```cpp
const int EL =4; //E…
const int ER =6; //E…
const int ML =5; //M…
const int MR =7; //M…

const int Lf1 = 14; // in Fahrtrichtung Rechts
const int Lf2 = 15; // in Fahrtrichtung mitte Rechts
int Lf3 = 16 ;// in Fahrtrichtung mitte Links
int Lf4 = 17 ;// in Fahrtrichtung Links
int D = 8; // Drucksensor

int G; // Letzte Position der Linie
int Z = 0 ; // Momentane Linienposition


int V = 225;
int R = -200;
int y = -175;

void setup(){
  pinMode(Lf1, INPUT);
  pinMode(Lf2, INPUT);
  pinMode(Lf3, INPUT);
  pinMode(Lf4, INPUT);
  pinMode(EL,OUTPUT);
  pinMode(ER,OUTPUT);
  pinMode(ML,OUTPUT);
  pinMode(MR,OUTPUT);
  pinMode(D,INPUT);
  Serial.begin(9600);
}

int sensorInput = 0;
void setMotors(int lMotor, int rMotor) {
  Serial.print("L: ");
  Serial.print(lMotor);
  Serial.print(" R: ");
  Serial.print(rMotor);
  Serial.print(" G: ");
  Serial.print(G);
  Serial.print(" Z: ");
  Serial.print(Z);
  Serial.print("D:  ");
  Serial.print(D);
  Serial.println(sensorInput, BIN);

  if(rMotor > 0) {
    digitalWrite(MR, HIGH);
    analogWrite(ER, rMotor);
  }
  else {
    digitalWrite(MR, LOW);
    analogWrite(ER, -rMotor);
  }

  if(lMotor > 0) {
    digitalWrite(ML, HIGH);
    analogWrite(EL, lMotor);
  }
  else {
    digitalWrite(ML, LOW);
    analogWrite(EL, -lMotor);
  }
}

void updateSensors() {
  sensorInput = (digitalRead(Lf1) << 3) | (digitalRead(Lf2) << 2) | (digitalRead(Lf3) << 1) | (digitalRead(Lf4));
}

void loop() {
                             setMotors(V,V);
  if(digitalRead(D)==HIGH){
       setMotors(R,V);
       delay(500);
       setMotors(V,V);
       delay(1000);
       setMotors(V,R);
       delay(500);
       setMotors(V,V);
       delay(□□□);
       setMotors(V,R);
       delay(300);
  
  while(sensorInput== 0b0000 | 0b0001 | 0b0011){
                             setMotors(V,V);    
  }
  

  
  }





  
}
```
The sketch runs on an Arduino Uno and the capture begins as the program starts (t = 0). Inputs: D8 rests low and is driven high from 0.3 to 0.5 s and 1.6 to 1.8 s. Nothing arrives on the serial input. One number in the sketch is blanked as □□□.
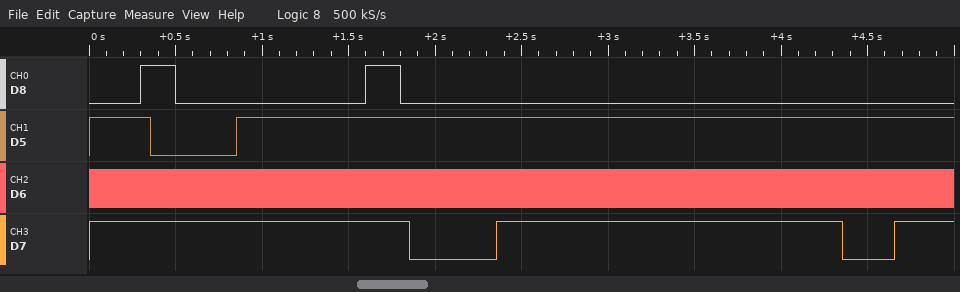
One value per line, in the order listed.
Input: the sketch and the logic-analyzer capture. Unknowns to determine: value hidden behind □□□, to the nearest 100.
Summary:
2000
